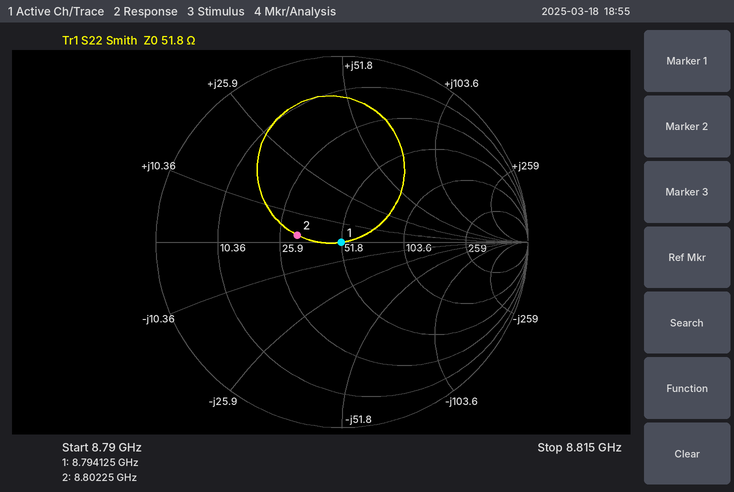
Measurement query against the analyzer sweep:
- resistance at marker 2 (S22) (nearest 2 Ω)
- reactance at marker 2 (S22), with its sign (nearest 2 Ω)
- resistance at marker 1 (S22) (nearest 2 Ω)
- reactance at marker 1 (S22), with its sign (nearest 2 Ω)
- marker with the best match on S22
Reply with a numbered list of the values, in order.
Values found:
1. 32 Ω
2. +2 Ω
3. 52 Ω
4. 0 Ω
5. marker 1
